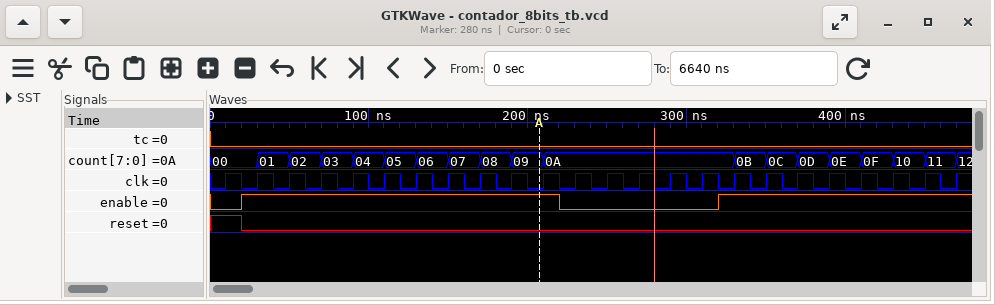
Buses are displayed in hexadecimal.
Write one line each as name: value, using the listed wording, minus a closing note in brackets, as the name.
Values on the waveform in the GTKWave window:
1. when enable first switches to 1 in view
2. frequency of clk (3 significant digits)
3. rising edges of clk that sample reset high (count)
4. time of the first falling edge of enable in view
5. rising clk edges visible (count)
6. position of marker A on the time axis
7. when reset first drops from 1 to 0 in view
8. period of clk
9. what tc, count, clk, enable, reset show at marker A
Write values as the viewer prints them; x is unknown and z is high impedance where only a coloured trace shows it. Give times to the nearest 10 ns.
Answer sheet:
when enable first switches to 1 in view: 20 ns
frequency of clk: 50.0 MHz
rising edges of clk that sample reset high: 1
time of the first falling edge of enable in view: 220 ns
rising clk edges visible: 24
position of marker A on the time axis: 210 ns
when reset first drops from 1 to 0 in view: 20 ns
period of clk: 20 ns
what tc, count, clk, enable, reset show at marker A: tc=0, count=09, clk=0, enable=1, reset=0
